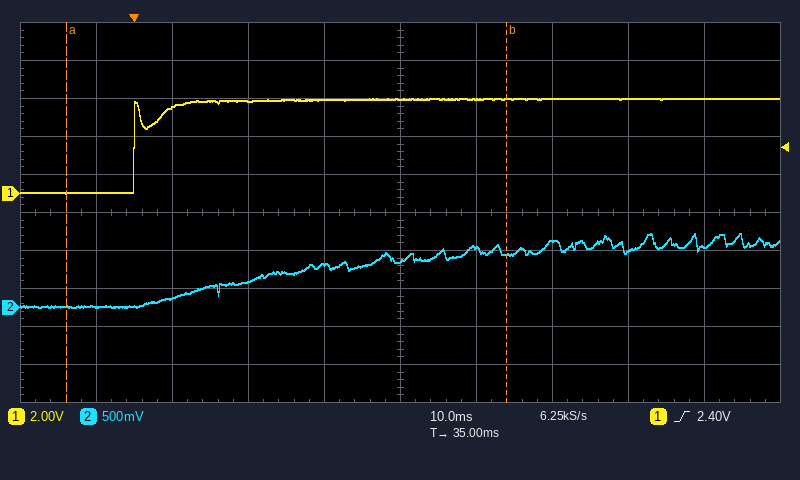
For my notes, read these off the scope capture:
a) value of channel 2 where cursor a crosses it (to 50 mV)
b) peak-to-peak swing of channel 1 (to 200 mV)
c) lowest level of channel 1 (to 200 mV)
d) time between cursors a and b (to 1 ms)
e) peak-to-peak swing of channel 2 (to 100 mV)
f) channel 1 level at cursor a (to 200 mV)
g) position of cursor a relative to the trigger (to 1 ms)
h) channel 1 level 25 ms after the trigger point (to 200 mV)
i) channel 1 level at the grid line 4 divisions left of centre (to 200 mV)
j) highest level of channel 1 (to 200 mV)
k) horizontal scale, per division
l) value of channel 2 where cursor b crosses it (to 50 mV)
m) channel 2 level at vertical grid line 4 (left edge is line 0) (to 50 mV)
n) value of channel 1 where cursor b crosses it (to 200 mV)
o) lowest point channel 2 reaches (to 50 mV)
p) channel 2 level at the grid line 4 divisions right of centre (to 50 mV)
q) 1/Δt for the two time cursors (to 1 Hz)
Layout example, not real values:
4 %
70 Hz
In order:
0 mV
5.0 V
0.0 V
58 ms
1.00 V
0.0 V
-9 ms
5.0 V
0.0 V
5.0 V
10 ms
700 mV
550 mV
5.0 V
0 mV
800 mV
17 Hz
